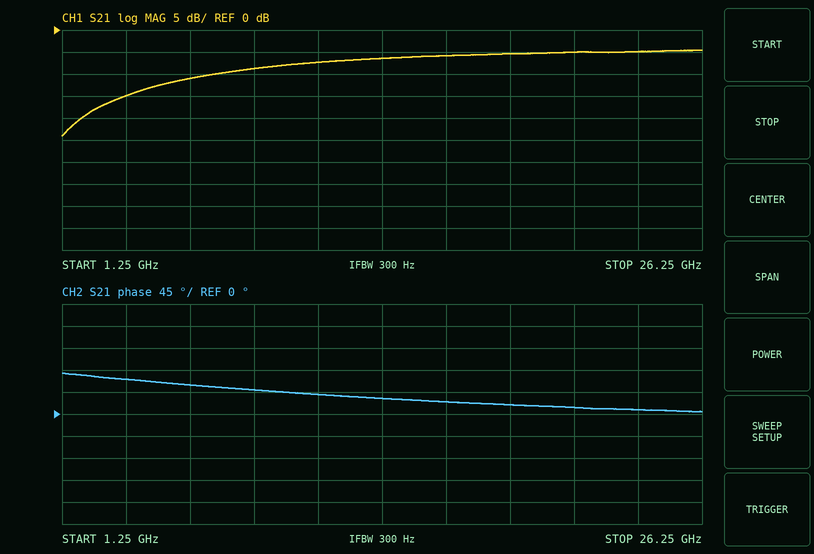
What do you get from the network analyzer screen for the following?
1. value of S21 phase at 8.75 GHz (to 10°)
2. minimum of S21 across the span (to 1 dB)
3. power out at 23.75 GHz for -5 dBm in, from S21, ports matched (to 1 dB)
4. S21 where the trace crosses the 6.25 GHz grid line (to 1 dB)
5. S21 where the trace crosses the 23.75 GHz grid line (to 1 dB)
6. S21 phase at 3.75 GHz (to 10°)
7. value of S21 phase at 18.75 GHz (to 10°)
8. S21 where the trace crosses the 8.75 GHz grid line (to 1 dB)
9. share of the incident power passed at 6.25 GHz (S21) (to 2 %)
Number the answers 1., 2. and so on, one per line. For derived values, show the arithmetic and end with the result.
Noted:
1. 50°
2. -24 dB
3. -5 dBm + (-5 dB) = -10 dBm
4. -11 dB
5. -5 dB
6. 70°
7. 20°
8. -9 dB
9. 10^(-11/10) ≈ 8 %
